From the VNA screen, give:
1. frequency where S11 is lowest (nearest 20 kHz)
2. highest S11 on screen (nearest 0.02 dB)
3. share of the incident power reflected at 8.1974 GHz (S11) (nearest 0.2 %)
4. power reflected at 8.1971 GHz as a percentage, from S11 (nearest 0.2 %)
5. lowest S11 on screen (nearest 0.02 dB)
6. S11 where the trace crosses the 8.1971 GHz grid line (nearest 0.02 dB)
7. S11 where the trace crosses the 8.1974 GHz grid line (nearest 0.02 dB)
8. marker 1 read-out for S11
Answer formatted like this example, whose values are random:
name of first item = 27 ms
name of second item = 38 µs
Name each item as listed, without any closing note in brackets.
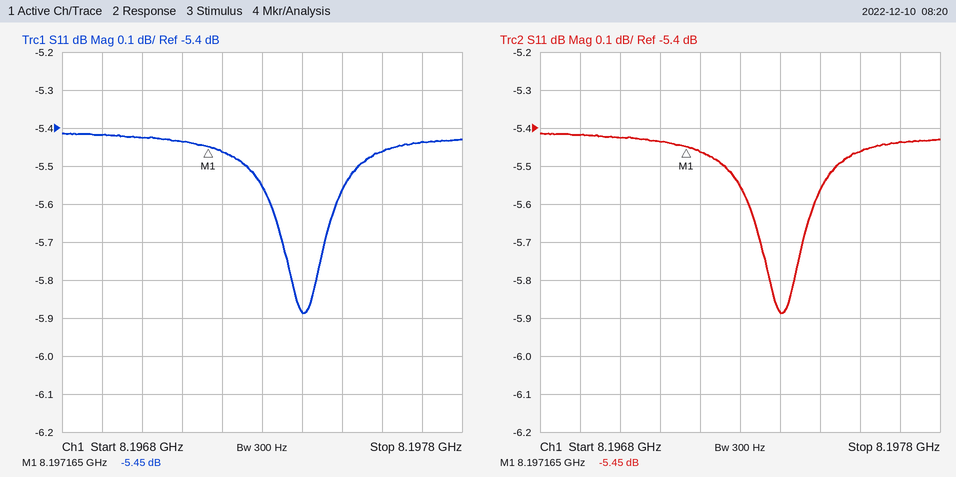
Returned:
frequency where S11 is lowest = 8.19740 GHz
highest S11 on screen = -5.42 dB
share of the incident power reflected at 8.1974 GHz (S11) = 25.8 %
power reflected at 8.1971 GHz as a percentage, from S11 = 28.6 %
lowest S11 on screen = -5.88 dB
S11 where the trace crosses the 8.1971 GHz grid line = -5.44 dB
S11 where the trace crosses the 8.1974 GHz grid line = -5.88 dB
marker 1 read-out for S11 = -5.45 dB
